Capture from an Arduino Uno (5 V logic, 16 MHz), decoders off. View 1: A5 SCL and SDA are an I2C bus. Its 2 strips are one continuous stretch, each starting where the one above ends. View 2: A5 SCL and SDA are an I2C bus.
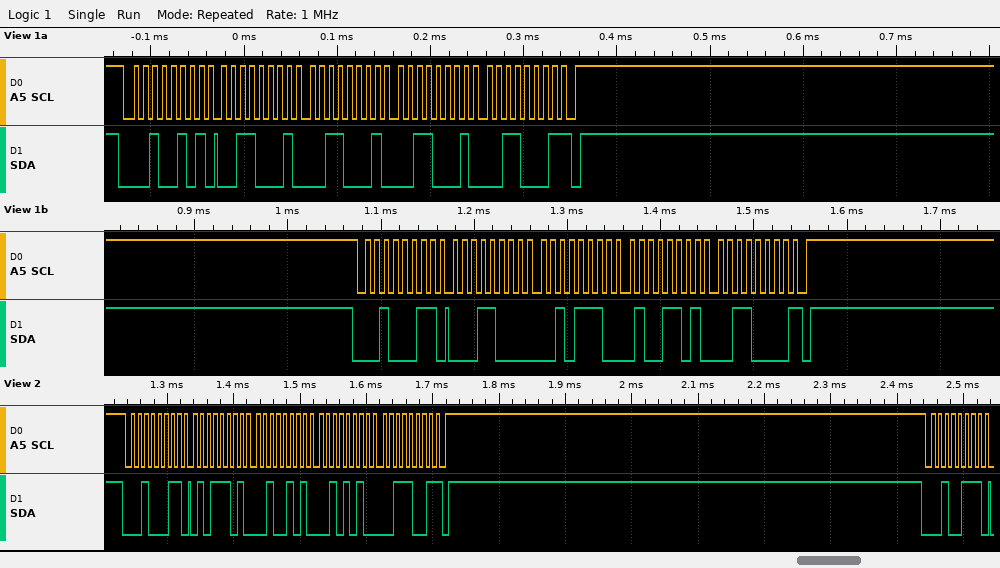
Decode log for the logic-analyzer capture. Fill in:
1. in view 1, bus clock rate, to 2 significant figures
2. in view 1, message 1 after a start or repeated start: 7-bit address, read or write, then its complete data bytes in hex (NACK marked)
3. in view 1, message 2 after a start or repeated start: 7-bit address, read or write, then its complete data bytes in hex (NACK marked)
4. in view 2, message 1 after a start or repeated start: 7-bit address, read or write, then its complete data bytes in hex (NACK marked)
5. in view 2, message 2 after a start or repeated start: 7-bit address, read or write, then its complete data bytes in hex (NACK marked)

100 kHz
0x12 read: 31 31 31 31 NACK
0x11 read: 18 2E 4D 30 NACK
0x11 read: 5D 25 2A 39 NACK
0x13 read
